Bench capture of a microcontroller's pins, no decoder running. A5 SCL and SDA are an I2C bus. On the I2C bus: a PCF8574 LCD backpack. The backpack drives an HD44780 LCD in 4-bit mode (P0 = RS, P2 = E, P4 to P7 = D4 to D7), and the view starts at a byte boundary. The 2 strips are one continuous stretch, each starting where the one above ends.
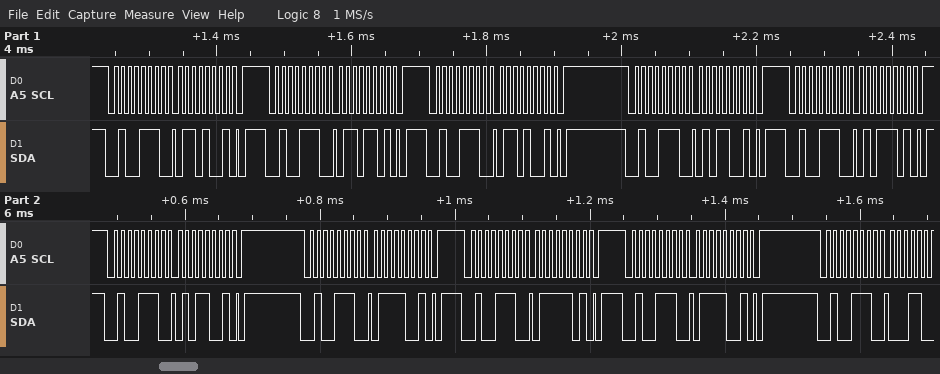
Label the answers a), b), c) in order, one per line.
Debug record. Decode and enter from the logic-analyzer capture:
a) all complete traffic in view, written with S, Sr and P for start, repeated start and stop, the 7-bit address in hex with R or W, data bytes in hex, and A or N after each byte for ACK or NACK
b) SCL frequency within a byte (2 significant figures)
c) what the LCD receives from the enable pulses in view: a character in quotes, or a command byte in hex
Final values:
a) S 27W A 69 A P S 27W A 6D A P S 27W A 69 A P S 27W A 59 A P S 27W A 5D A P S 27W A 59 A P S 27W A 79 A P S 27W A 7D A P S 27W A 79 A P S 27W A
b) 100 kHz
c) 'e'
